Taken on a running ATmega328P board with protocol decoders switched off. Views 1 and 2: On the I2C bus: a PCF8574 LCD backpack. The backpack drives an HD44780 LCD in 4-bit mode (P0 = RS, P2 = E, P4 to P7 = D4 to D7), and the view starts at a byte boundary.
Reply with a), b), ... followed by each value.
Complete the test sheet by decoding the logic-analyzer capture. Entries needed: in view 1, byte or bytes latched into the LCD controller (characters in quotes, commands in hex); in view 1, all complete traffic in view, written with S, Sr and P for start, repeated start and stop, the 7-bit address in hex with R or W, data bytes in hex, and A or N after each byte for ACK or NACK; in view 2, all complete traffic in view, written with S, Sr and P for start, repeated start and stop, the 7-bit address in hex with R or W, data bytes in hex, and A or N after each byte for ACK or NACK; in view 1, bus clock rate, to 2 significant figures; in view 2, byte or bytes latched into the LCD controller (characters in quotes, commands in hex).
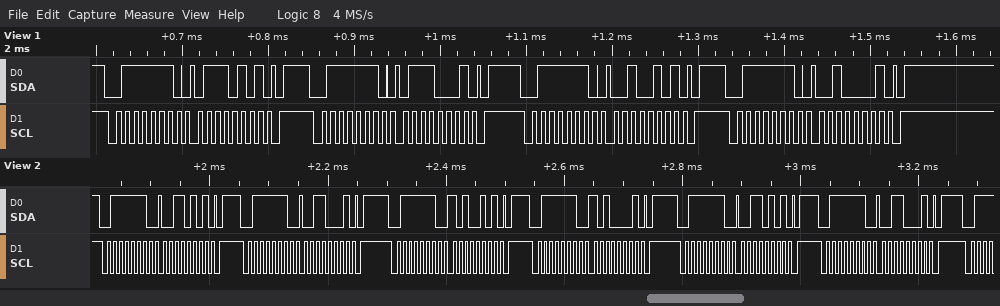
a) 'r'
b) S 3FW A 75 A P S 3FW A 71 A P S 3FW A 25 A P S 3FW A 21 A P
c) S 3FW A 35 A P S 3FW A 31 A P S 3FW A A5 A P S 3FW A A1 A P S 3FW A 35 A P S 3FW A 31 A P
d) 100 kHz
e) ':'
